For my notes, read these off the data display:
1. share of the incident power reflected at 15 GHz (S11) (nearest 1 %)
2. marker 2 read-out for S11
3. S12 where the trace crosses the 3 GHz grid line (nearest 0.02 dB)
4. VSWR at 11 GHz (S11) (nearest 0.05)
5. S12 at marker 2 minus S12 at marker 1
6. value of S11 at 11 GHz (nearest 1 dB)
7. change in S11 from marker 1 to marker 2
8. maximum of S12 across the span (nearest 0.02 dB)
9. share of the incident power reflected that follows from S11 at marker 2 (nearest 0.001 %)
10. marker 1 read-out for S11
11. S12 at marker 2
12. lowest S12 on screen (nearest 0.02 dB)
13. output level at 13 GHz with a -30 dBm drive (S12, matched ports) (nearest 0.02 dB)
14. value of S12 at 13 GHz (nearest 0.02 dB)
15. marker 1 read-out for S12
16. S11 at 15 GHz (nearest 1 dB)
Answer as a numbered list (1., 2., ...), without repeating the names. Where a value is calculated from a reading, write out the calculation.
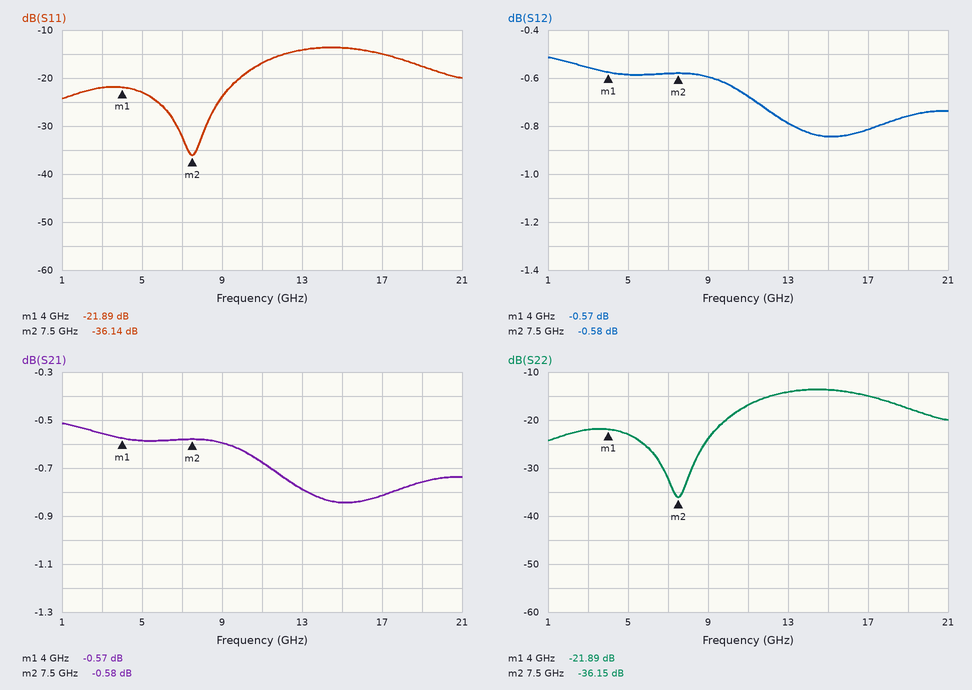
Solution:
1. 10^(-14/10) ≈ 4 %
2. -36.14 dB
3. -0.56 dB
4. |Γ| = 10^(-17/20) = 0.1413; VSWR = (1 + 0.1413)/(1 − 0.1413) ≈ 1.33, so 1.35 to the nearest 0.05
5. -0.58 − (-0.57) = -0.01 dB
6. -17 dB
7. -36.14 − (-21.89) = -14.25 dB
8. -0.52 dB
9. 10^(-36.14/10) ≈ 0.024 %
10. -21.89 dB
11. -0.58 dB
12. -0.84 dB
13. -30 dBm + (-0.78 dB) = -30.78 dBm
14. -0.78 dB
15. -0.57 dB
16. -14 dB
